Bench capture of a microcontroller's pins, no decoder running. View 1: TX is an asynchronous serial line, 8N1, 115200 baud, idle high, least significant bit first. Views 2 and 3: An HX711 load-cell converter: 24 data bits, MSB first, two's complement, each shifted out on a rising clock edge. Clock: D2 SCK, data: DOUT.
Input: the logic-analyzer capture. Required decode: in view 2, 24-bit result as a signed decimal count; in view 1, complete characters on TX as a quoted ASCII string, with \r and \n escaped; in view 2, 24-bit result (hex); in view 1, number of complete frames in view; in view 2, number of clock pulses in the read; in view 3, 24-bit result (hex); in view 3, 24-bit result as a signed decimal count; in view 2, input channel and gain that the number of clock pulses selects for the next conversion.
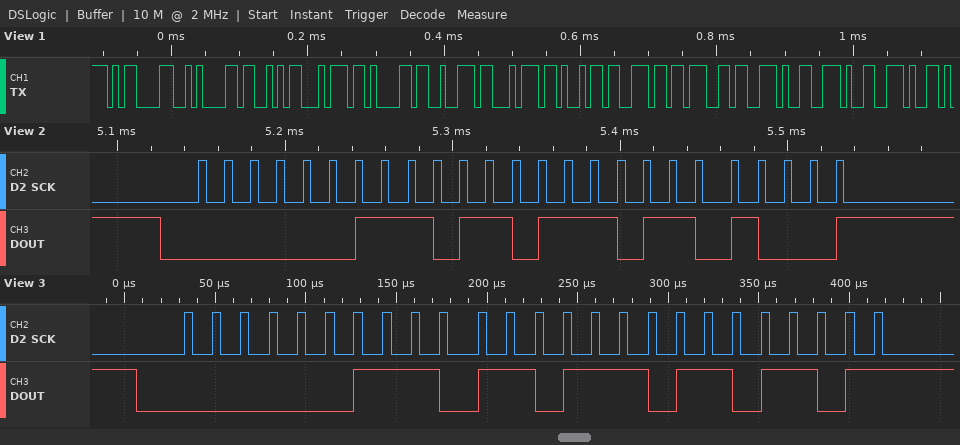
243560
"\r\nStarting..."
0x03B768
13
25
0x03B76D
243565
channel A, gain 128
